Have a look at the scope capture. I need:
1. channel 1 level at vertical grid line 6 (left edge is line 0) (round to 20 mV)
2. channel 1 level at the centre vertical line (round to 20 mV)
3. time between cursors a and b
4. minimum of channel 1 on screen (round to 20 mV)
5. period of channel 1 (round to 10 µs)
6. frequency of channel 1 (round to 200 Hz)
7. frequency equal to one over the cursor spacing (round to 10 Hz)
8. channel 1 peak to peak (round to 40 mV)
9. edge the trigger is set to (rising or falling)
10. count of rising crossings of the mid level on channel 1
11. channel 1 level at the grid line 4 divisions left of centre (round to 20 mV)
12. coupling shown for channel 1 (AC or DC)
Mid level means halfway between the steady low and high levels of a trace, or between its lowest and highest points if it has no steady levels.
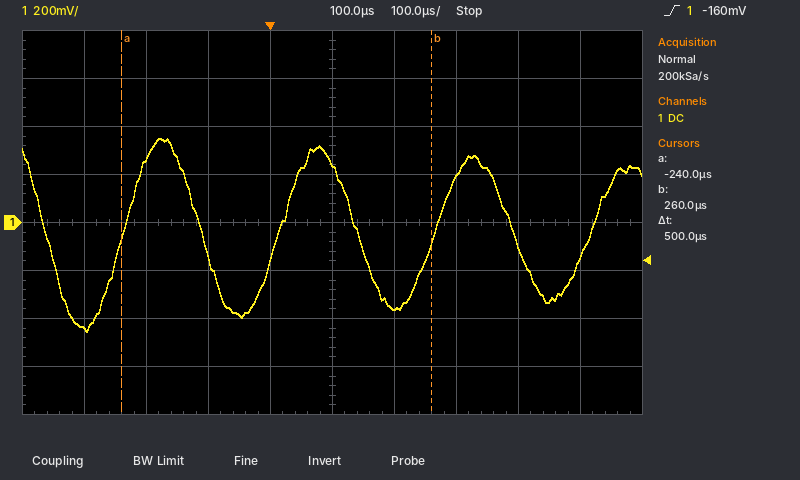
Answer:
-360 mV
240 mV
500 µs
-460 mV
250 µs
4.0 kHz
2.00 kHz
800 mV
rising
4
-440 mV
DC
